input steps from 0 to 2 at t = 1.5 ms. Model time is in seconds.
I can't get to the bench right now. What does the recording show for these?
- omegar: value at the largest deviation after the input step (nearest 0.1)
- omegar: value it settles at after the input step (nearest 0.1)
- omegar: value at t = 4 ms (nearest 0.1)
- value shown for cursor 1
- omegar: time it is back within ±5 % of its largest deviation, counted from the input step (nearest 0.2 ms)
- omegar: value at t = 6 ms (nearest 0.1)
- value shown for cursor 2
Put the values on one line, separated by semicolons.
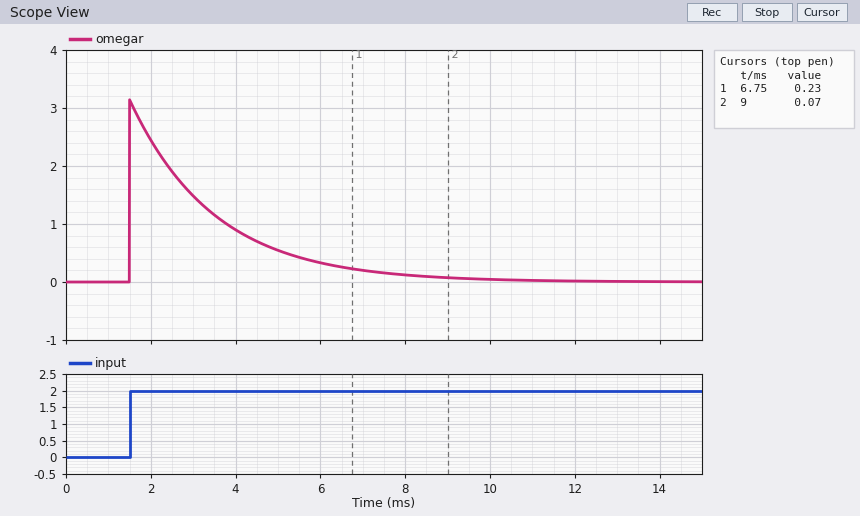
3.1; 0.0; 0.9; 0.23; 6.0 ms; 0.3; 0.07
